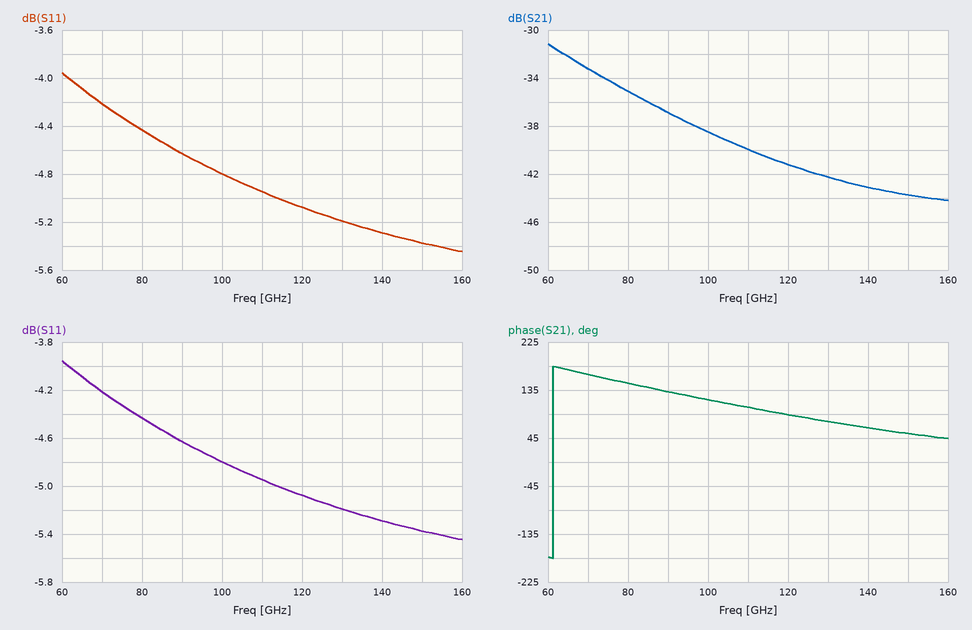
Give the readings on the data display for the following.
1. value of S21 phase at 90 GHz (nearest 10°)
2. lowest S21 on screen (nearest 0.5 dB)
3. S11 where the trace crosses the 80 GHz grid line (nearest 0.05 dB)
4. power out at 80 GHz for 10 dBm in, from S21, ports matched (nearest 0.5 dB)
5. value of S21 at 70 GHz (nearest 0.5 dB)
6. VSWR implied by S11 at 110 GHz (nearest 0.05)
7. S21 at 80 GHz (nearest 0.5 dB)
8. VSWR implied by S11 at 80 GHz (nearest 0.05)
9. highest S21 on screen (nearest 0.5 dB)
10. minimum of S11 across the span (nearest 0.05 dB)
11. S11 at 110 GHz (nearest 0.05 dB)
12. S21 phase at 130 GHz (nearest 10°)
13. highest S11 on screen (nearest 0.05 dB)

130°
-44.0 dB
-4.45 dB
-25.0 dBm
-33.0 dB
3.60
-35.0 dB
4.00
-31.0 dB
-5.45 dB
-4.95 dB
80°
-3.95 dB
